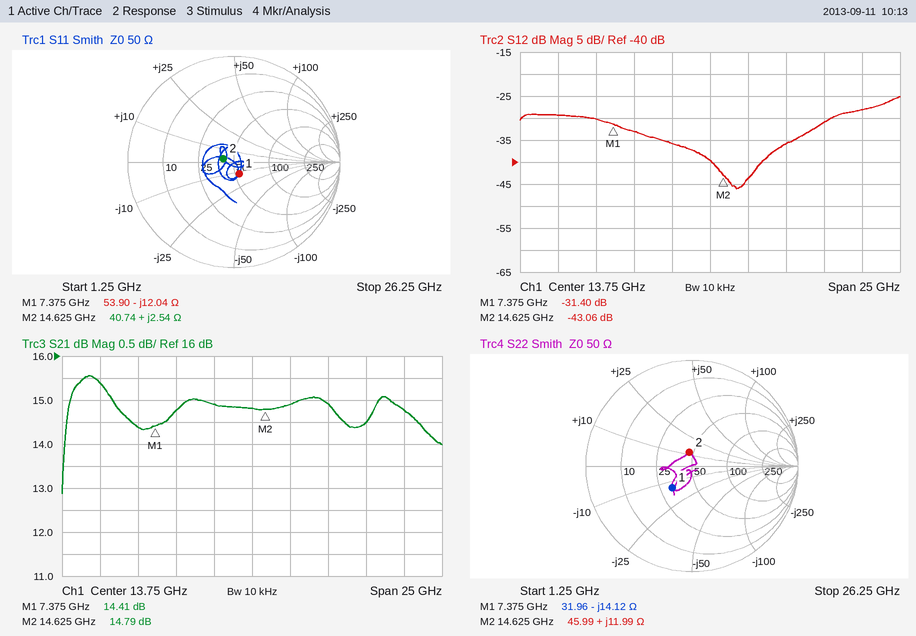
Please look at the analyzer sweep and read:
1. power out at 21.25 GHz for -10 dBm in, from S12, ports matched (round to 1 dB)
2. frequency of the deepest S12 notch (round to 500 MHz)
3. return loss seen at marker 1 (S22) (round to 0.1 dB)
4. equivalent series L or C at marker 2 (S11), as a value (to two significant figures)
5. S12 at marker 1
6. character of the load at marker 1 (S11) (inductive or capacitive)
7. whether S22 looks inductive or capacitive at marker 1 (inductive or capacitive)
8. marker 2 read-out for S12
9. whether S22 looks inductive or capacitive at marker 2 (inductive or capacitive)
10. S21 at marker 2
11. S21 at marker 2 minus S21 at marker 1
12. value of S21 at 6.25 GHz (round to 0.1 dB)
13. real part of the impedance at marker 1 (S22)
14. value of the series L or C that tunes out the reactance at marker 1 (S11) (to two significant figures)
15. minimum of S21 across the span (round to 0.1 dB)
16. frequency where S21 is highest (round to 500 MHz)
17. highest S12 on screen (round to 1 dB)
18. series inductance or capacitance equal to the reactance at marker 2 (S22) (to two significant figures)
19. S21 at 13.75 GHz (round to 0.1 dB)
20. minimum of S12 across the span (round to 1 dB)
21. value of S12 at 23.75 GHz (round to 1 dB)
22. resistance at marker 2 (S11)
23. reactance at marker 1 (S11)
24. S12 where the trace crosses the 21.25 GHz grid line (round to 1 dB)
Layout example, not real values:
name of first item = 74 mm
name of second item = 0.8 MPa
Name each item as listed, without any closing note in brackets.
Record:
power out at 21.25 GHz for -10 dBm in, from S12, ports matched = -41 dBm
frequency of the deepest S12 notch = 15.5 GHz
return loss seen at marker 1 (S22) = 11.2 dB
equivalent series L or C at marker 2 (S11), as a value = 28 pH
S12 at marker 1 = -31.40 dB
character of the load at marker 1 (S11) = capacitive
whether S22 looks inductive or capacitive at marker 1 = capacitive
marker 2 read-out for S12 = -43.06 dB
whether S22 looks inductive or capacitive at marker 2 = inductive
S21 at marker 2 = 14.79 dB
S21 at marker 2 minus S21 at marker 1 = 0.38 dB
value of S21 at 6.25 GHz = 14.4 dB
real part of the impedance at marker 1 = 31.96 Ω
value of the series L or C that tunes out the reactance at marker 1 (S11) = 260 pH
minimum of S21 across the span = 12.9 dB
frequency where S21 is highest = 3.0 GHz
highest S12 on screen = -25 dB
series inductance or capacitance equal to the reactance at marker 2 (S22) = 130 pH
S21 at 13.75 GHz = 14.8 dB
minimum of S12 across the span = -46 dB
value of S12 at 23.75 GHz = -28 dB
resistance at marker 2 = 40.74 Ω
reactance at marker 1 = -12.04 Ω
S12 where the trace crosses the 21.25 GHz grid line = -31 dB
